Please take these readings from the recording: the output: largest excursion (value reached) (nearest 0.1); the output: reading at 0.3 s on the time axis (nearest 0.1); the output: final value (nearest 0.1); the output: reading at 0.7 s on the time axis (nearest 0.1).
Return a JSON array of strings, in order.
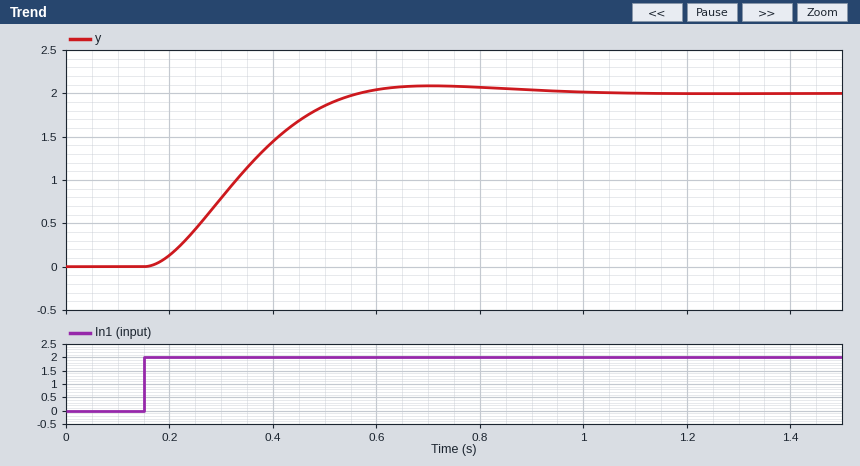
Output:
["2.1", "0.8", "2.0", "2.1"]
